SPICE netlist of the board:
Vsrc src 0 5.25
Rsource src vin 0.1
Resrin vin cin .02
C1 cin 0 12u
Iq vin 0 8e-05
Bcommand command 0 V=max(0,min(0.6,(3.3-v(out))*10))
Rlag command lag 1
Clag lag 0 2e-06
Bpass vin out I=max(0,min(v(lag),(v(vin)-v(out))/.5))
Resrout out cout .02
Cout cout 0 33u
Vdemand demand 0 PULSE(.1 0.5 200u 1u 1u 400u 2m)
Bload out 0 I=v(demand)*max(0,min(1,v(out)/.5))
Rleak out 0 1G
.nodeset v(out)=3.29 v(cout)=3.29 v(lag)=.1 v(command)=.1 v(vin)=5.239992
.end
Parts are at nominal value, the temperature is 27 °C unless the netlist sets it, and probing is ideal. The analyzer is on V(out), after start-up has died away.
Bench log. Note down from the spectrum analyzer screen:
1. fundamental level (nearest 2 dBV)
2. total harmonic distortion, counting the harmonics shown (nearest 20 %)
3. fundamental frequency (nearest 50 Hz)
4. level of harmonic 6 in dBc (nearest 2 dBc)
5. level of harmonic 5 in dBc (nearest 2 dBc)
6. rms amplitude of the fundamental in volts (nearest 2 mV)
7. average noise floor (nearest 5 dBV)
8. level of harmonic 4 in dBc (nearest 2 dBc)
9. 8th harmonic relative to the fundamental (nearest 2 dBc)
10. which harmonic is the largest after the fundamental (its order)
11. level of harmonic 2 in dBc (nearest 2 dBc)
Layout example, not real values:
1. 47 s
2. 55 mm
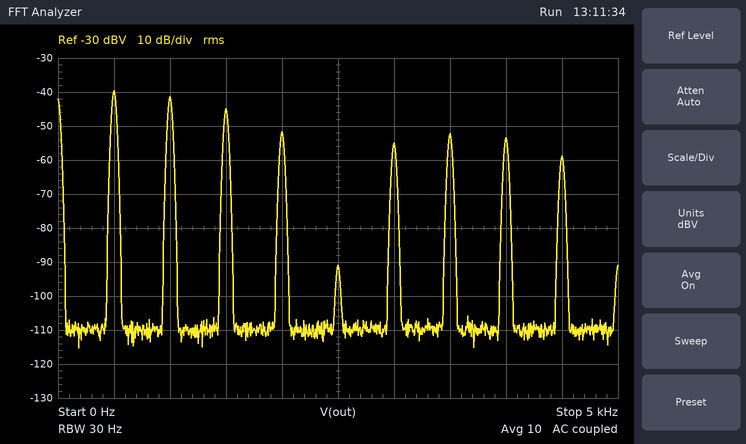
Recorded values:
1. -40 dBV
2. 100 %
3. 500 Hz
4. -16 dBc
5. -52 dBc
6. 10 mV
7. -110 dBV
8. -12 dBc
9. -14 dBc
10. 2
11. -2 dBc
